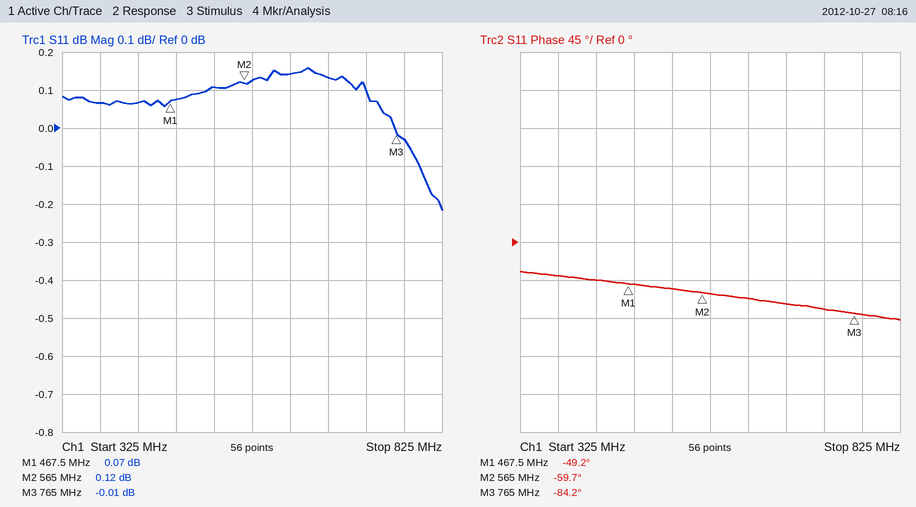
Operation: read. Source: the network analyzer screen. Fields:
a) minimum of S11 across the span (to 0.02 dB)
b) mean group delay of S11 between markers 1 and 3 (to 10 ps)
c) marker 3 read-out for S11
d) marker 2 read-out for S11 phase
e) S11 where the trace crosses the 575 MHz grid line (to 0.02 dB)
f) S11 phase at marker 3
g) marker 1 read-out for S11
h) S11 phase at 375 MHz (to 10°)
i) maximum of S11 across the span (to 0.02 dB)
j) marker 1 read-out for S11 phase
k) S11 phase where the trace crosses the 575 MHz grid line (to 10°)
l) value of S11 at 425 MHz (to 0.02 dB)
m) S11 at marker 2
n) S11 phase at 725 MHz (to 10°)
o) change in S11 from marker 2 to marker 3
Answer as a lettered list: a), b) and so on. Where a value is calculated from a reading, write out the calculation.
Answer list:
a) -0.22 dB
b) −(-84.2° − (-49.2°))/(360° × 297.5 MHz) ≈ 327 ps, so 330 ps to the nearest 10 ps
c) -0.01 dB
d) -59.7°
e) 0.12 dB
f) -84.2°
g) 0.07 dB
h) -40°
i) 0.16 dB
j) -49.2°
k) -60°
l) 0.06 dB
m) 0.12 dB
n) -80°
o) -0.01 − (0.12) = -0.13 dB
